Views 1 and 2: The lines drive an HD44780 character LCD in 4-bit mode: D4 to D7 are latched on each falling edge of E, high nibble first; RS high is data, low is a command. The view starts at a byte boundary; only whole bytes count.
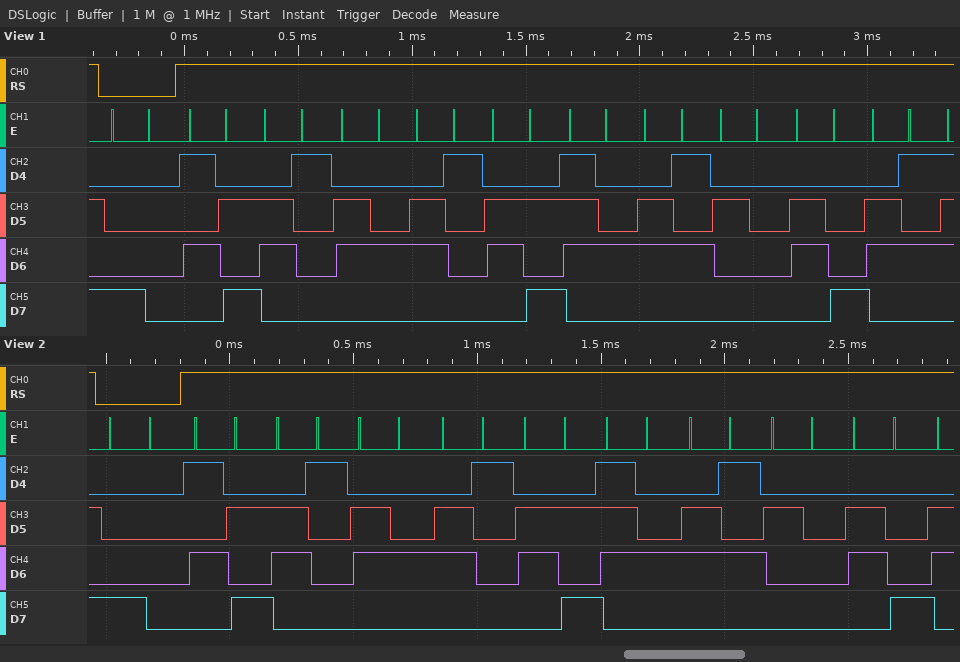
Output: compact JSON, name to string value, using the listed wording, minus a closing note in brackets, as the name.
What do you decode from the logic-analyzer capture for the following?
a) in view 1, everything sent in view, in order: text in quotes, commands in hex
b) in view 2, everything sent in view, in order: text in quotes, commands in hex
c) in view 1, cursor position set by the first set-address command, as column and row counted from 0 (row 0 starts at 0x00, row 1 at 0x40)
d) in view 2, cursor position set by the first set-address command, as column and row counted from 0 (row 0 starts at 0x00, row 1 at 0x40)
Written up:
{"in view 1, everything sent in view, in order: text in quotes, commands in hex": "0x80 \"Zadajte he\"", "in view 2, everything sent in view, in order: text in quotes, commands in hex": "0x80 \"Zadajte h\"", "in view 1, cursor position set by the first set-address command, as column and row counted from 0": "column 0, row 0", "in view 2, cursor position set by the first set-address command, as column and row counted from 0": "column 0, row 0"}
